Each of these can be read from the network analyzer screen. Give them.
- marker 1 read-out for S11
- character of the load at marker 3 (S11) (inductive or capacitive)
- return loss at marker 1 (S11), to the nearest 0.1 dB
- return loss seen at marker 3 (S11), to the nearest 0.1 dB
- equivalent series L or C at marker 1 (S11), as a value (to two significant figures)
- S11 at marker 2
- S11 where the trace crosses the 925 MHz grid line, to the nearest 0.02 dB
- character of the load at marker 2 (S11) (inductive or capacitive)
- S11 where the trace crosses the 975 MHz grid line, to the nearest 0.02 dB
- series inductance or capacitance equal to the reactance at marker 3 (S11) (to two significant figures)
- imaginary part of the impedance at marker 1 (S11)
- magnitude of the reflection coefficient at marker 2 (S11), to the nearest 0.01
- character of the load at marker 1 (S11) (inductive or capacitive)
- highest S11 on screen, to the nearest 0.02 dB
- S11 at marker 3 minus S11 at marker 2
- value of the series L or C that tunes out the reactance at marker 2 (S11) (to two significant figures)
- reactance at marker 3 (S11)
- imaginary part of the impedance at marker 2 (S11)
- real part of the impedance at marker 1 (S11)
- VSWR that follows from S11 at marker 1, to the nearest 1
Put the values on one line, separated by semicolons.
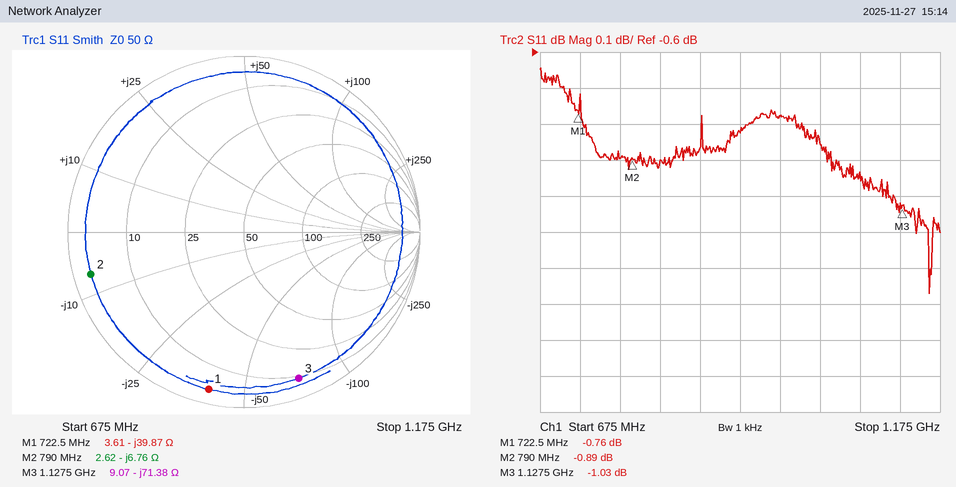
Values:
-0.76 dB; capacitive; 0.8 dB; 1.0 dB; 5.5 pF; -0.89 dB; -0.82 dB; capacitive; -0.78 dB; 2.0 pF; -39.87 Ω; 0.90; capacitive; -0.64 dB; -0.14 dB; 1.4 nH; -71.38 Ω; -6.76 Ω; 3.61 Ω; 23
